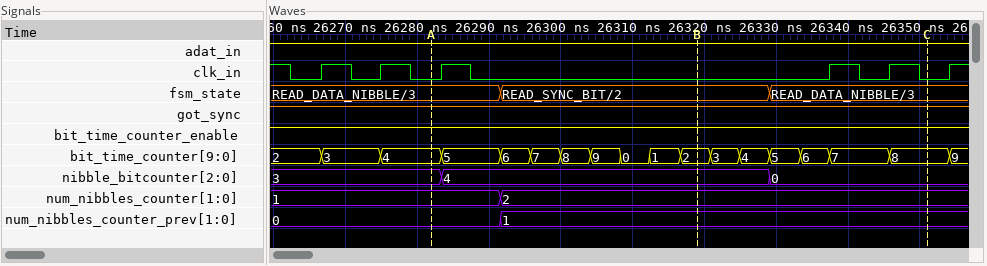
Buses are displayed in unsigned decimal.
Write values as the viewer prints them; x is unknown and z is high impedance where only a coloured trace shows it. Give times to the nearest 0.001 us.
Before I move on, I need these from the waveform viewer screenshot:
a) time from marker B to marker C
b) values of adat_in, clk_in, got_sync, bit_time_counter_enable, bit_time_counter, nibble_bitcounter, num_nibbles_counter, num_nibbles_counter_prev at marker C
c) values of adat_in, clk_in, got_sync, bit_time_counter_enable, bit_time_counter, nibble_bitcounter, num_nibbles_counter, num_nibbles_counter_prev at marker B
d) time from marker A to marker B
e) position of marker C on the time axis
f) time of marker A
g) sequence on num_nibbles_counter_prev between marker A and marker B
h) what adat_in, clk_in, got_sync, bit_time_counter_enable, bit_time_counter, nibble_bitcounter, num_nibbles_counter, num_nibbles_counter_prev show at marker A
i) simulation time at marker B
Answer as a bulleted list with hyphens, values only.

- 0.032 us
- adat_in=1, clk_in=0, got_sync=1, bit_time_counter_enable=1, bit_time_counter=8, nibble_bitcounter=0, num_nibbles_counter=2, num_nibbles_counter_prev=1
- adat_in=1, clk_in=0, got_sync=1, bit_time_counter_enable=1, bit_time_counter=2, nibble_bitcounter=4, num_nibbles_counter=2, num_nibbles_counter_prev=1
- 0.037 us
- 26.351 us
- 26.282 us
- 0, 1
- adat_in=1, clk_in=0, got_sync=1, bit_time_counter_enable=1, bit_time_counter=4, nibble_bitcounter=3, num_nibbles_counter=1, num_nibbles_counter_prev=0
- 26.319 us
